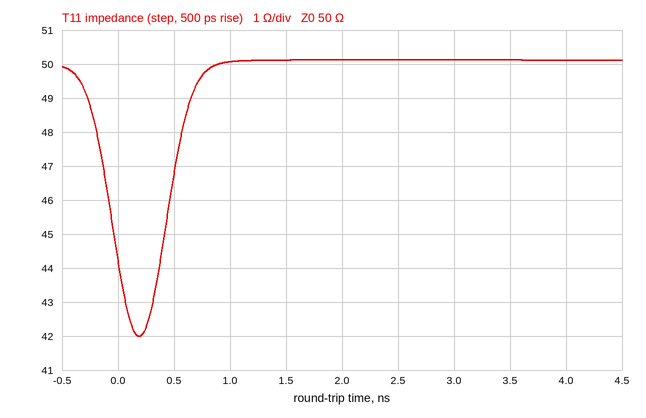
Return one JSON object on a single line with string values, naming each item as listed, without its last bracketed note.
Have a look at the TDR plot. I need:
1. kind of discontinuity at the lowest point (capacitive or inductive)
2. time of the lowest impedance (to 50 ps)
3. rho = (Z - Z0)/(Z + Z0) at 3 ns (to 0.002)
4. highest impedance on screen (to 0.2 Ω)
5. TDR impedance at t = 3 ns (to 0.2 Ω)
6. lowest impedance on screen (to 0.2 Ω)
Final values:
{"kind of discontinuity at the lowest point": "capacitive", "time of the lowest impedance": "200 ps", "rho = (Z - Z0)/(Z + Z0) at 3 ns": "+0.002", "highest impedance on screen": "50.2 Ω", "TDR impedance at t = 3 ns": "50.2 Ω", "lowest impedance on screen": "42.0 Ω"}
